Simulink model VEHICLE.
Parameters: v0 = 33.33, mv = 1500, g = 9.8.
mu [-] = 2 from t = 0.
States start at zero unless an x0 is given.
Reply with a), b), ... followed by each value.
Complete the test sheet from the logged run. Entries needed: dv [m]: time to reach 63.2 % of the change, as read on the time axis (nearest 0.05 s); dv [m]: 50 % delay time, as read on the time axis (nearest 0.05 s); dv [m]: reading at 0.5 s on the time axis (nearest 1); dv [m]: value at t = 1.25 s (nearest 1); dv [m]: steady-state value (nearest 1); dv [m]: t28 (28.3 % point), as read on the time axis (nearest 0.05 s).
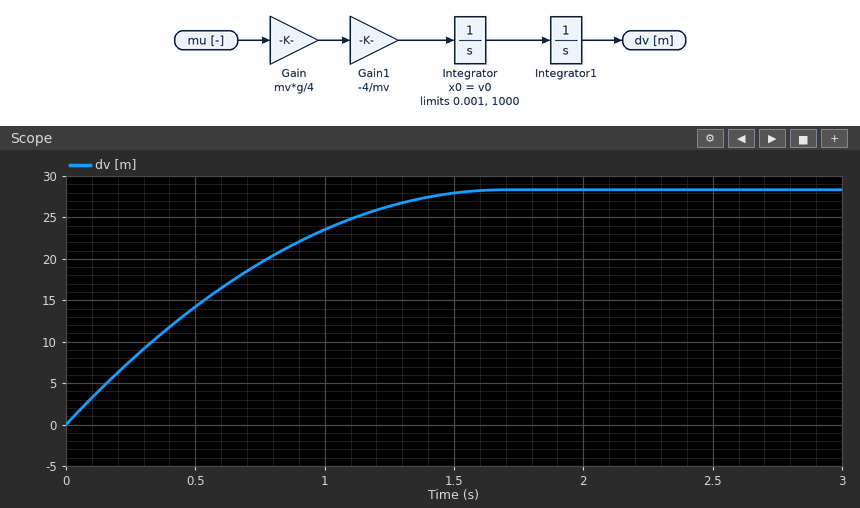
a) 0.65 s
b) 0.50 s
c) 14
d) 26
e) 28
f) 0.25 s
